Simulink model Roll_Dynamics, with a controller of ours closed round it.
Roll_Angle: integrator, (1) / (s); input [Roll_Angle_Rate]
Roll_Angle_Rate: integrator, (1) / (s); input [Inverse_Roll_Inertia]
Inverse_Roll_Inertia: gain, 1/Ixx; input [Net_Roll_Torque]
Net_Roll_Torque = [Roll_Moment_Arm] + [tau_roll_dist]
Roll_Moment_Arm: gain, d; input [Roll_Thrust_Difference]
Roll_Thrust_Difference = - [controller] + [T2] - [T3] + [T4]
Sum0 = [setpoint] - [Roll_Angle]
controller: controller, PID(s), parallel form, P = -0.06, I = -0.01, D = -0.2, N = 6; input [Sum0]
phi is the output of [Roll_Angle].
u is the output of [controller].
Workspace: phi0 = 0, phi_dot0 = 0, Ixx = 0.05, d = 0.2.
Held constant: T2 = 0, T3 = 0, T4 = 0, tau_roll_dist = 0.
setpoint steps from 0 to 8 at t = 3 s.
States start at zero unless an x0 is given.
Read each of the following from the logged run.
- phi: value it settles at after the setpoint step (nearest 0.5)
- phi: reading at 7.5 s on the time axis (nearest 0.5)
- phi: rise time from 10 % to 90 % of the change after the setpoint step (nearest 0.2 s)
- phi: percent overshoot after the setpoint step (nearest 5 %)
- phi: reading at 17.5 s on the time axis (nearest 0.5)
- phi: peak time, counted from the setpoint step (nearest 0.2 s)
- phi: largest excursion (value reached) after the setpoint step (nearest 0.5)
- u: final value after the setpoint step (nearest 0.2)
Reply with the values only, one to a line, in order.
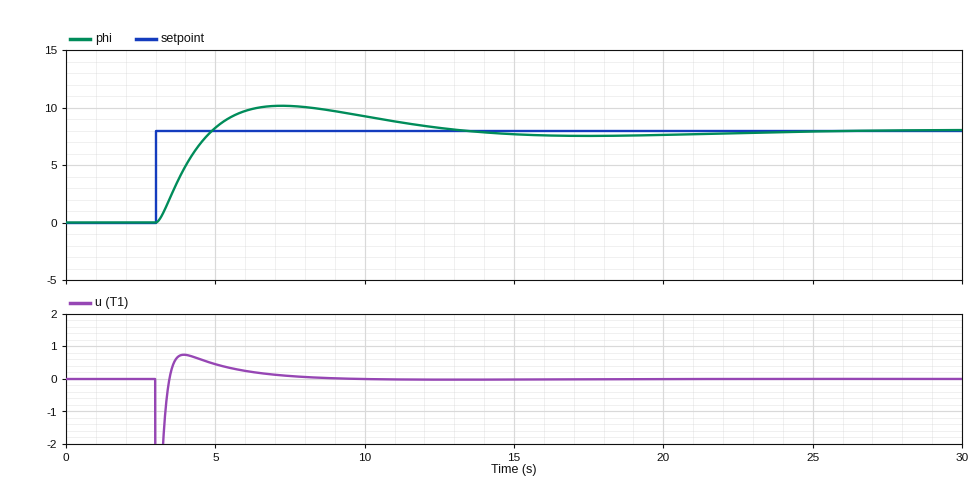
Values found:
8.0
10.0
1.4 s
25 %
7.5
4.2 s
10.0
0.0
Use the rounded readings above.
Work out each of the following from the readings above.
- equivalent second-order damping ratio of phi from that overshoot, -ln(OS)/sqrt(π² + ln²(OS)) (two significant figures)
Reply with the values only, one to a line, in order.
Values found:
0.40
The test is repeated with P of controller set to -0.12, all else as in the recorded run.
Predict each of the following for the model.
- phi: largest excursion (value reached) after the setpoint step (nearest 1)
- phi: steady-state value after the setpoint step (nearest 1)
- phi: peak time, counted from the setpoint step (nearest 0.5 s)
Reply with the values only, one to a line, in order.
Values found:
11
8
3.0 s
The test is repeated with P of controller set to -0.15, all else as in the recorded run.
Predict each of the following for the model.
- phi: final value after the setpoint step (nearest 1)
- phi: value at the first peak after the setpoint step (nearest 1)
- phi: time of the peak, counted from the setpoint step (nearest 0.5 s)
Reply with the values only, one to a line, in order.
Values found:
8
11
3.0 s
